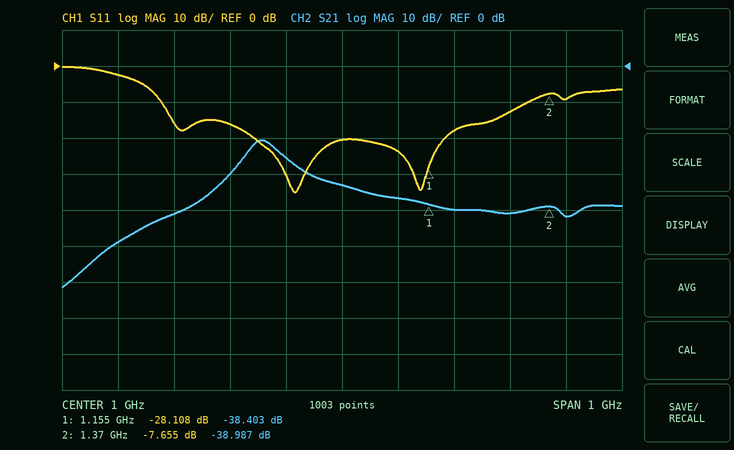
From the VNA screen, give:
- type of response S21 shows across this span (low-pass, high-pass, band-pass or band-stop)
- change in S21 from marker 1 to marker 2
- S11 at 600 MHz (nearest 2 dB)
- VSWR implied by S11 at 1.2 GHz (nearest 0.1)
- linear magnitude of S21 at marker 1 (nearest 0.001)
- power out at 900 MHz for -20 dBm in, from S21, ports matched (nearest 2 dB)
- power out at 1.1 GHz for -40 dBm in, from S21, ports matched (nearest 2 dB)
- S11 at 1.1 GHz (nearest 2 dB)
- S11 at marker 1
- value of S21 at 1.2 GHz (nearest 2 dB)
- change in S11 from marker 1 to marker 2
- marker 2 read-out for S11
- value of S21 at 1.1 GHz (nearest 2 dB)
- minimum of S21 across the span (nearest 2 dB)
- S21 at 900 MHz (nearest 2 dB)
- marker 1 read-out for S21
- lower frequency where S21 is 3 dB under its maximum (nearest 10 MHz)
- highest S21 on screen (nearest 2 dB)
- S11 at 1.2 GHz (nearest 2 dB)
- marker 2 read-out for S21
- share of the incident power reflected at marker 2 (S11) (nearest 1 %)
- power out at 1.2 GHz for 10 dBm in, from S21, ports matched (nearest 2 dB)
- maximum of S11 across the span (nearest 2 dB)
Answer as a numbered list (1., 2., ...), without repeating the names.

1. band-pass
2. -0.584 dB
3. -2 dB
4. 1.3
5. 0.012
6. -46 dBm
7. -76 dBm
8. -24 dB
9. -28.108 dB
10. -40 dB
11. 20.453 dB
12. -7.655 dB
13. -36 dB
14. -62 dB
15. -26 dB
16. -38.403 dB
17. 830 MHz
18. -20 dB
19. -18 dB
20. -38.987 dB
21. 17 %
22. -30 dBm
23. 0 dB
